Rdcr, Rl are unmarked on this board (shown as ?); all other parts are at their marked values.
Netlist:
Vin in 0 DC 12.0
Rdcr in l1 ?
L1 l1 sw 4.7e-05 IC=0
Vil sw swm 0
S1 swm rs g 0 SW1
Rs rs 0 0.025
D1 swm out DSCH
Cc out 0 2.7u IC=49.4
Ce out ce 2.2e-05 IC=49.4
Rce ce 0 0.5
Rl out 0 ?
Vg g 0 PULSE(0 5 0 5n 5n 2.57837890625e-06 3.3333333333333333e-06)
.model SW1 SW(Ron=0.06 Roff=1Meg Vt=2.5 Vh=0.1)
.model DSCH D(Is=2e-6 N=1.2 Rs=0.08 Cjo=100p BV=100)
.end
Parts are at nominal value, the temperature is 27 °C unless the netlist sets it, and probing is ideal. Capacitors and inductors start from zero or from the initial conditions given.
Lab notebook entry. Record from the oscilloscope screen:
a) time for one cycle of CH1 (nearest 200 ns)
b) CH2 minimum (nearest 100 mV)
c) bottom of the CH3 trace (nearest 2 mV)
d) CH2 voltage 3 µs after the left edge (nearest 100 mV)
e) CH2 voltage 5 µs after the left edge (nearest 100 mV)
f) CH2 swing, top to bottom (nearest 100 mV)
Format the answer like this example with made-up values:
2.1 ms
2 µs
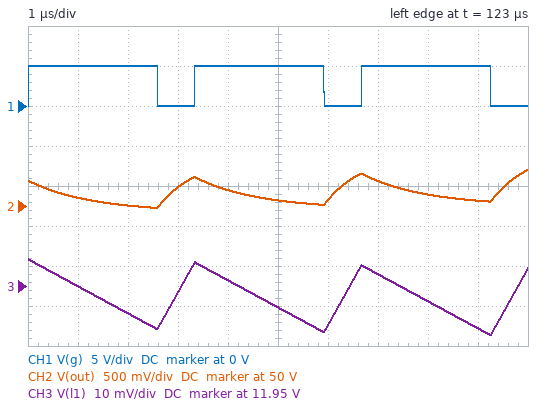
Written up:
3.4 µs
50.0 V
11.938 V
50.2 V
50.1 V
500 mV
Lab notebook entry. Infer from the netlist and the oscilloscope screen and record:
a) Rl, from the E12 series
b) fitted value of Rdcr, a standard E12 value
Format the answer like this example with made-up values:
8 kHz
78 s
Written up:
330 Ω
0.027 Ω
